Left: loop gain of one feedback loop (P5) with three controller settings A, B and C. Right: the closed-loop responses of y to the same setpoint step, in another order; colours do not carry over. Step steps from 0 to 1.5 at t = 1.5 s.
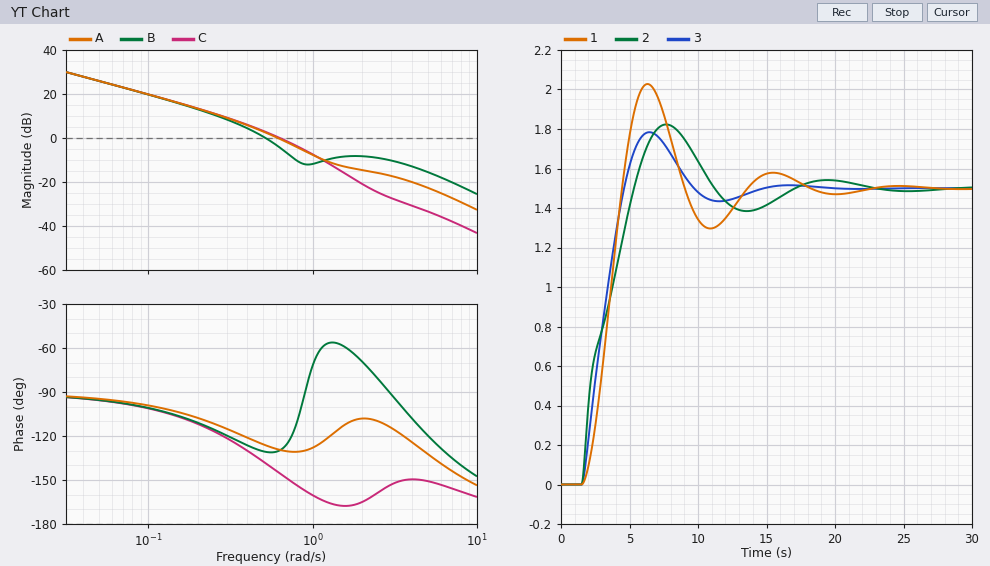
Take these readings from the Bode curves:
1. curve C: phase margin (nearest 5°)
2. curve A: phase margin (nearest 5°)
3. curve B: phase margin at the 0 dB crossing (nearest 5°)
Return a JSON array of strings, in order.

["35°", "50°", "50°"]
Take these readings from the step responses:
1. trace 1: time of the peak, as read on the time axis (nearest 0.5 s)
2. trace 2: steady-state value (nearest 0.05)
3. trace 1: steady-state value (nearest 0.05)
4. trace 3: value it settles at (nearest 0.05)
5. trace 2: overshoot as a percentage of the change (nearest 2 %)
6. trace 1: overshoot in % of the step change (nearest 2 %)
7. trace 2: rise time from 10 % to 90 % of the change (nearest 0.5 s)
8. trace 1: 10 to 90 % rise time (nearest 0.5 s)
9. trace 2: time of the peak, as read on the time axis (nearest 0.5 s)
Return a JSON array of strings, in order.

["6.5 s", "1.50", "1.50", "1.50", "22 %", "36 %", "3.0 s", "2.0 s", "7.5 s"]
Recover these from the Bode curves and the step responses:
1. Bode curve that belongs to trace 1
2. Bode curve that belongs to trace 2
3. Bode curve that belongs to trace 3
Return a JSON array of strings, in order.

["C", "B", "A"]
